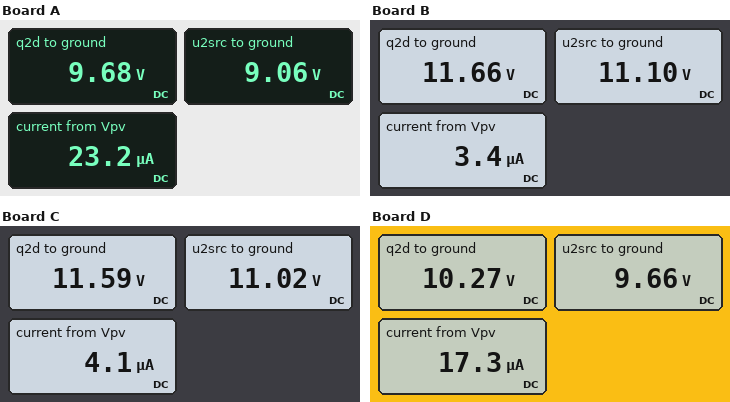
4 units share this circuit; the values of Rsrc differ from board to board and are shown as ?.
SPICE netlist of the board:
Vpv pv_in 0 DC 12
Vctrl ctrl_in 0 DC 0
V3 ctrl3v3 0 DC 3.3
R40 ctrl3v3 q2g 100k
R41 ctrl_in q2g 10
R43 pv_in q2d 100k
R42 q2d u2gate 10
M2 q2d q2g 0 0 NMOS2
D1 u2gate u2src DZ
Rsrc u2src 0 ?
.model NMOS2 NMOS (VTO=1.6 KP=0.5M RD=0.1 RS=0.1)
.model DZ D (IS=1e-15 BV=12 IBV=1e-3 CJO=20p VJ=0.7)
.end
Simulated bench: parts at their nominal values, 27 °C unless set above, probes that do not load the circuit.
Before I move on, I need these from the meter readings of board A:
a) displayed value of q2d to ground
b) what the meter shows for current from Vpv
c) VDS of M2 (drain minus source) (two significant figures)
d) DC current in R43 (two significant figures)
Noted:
9.68 V
23.2 µA
9.7 V
23 µA
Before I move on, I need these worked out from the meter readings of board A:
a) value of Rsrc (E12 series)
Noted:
390 kΩ
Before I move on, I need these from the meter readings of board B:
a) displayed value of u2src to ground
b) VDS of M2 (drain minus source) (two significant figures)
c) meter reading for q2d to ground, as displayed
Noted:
11.10 V
12 V
11.66 V
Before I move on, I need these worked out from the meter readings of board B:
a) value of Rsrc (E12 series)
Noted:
3.3 MΩ
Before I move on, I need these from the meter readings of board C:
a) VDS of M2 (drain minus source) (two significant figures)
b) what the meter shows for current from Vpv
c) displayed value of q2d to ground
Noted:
12 V
4.1 µA
11.59 V
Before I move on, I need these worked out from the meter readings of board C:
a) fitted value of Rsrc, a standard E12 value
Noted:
2.7 MΩ
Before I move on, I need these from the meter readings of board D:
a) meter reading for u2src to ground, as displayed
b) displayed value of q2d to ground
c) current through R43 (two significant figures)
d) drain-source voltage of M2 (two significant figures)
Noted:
9.66 V
10.27 V
17 µA
10 V
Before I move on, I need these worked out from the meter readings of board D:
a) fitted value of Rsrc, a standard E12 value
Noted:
560 kΩ
